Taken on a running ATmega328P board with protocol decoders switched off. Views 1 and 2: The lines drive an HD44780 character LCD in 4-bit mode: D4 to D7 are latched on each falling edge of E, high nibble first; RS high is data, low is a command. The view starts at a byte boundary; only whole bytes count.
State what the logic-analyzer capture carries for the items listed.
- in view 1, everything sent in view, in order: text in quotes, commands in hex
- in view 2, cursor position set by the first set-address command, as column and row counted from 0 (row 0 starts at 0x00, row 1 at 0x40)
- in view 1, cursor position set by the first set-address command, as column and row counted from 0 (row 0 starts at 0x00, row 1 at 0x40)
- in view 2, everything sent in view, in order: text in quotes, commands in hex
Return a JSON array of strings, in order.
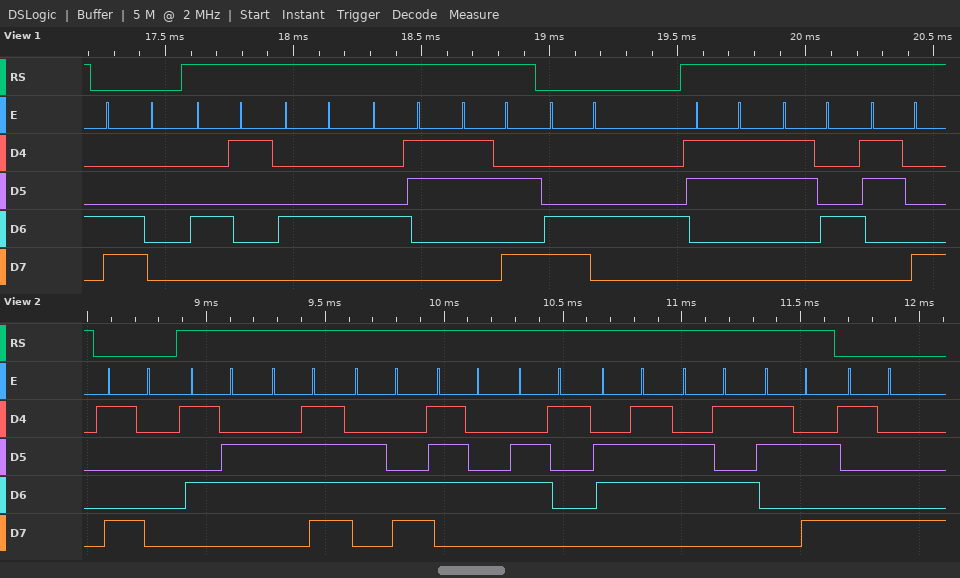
["0xC0 \"ADC:\" 0xC4 \"348\"", "column 16, row 0", "column 0, row 1", "0x90 \"Voltage:\" 0x98"]
